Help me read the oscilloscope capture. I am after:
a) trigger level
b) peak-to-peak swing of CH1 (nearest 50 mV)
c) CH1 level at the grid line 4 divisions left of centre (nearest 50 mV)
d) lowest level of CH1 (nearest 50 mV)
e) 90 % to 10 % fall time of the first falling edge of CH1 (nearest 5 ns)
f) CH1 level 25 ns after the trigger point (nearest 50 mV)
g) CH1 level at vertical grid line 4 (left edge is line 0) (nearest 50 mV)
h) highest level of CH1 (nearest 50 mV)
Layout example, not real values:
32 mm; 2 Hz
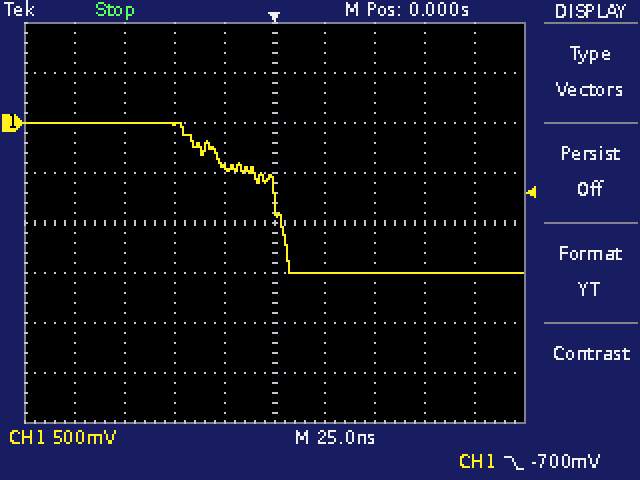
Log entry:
-700 mV; 1.50 V; 0 mV; -1.50 V; 50 ns; -1.50 V; -450 mV; 0 mV
